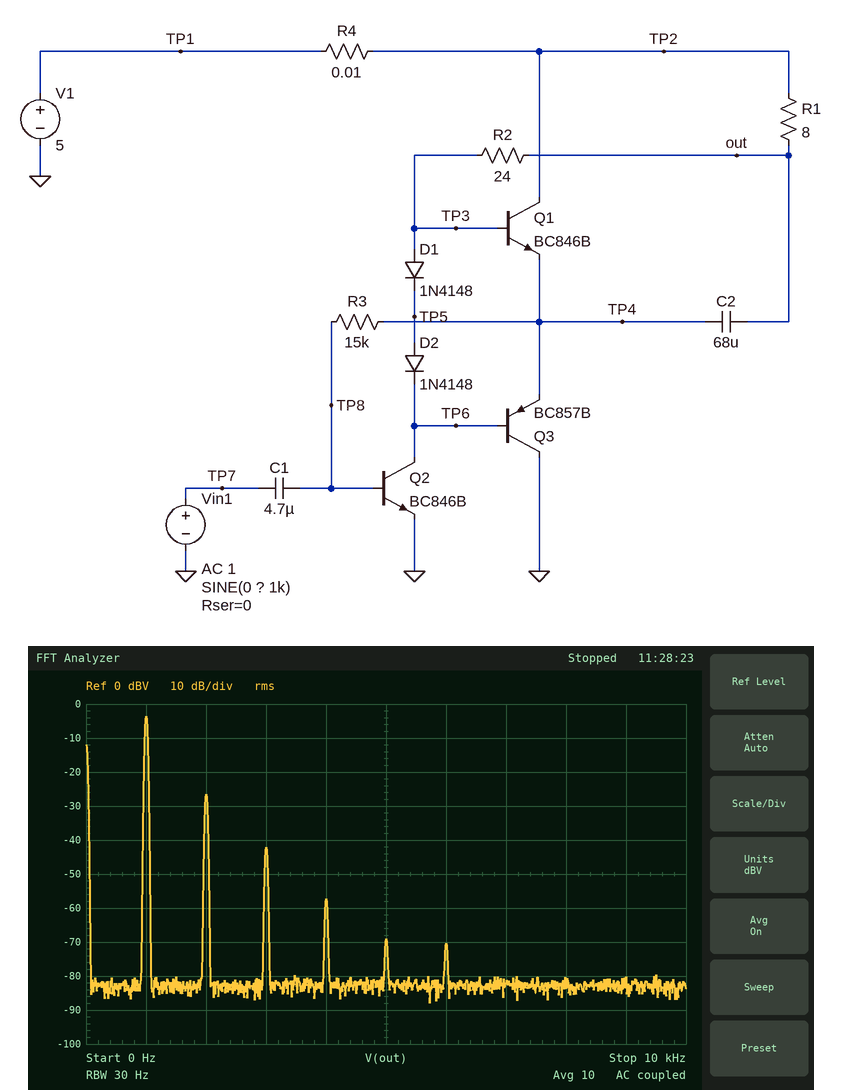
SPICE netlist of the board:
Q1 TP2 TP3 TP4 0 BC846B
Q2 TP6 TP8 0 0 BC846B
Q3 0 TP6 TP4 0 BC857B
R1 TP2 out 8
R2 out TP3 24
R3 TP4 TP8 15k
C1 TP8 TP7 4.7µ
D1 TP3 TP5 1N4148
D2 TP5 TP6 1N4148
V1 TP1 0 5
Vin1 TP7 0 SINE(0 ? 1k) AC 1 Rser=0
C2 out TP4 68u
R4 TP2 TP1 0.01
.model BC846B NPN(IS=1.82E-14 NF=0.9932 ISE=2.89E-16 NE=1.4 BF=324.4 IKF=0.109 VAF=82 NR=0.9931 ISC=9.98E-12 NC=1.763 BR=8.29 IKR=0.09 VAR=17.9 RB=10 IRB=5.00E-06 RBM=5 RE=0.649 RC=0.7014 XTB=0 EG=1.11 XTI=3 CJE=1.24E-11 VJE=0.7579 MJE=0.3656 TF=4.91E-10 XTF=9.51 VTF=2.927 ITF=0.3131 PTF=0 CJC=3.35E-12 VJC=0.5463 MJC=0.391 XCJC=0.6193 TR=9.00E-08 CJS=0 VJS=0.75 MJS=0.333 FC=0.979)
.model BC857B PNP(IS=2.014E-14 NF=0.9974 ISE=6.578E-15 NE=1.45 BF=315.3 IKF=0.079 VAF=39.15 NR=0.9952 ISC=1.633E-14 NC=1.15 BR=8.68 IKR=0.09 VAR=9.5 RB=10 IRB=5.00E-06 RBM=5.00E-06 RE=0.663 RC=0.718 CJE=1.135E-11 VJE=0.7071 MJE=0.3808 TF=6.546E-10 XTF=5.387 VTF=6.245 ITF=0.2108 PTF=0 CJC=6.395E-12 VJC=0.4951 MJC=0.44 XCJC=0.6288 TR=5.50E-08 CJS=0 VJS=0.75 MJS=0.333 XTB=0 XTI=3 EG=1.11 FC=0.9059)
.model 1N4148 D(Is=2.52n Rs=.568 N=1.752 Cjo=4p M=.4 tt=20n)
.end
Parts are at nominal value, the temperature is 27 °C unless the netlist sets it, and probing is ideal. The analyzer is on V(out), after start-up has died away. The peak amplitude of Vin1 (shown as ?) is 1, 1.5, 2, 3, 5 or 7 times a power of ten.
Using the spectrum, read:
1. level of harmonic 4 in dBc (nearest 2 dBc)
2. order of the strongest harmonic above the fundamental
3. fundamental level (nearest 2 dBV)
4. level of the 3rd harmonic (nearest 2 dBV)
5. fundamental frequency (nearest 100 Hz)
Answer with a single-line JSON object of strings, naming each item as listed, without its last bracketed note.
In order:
{"level of harmonic 4 in dBc": "-54 dBc", "order of the strongest harmonic above the fundamental": "2", "fundamental level": "-4 dBV", "level of the 3rd harmonic": "-42 dBV", "fundamental frequency": "1.0 kHz"}
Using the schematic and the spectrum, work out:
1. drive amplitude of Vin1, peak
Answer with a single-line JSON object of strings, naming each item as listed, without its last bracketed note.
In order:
{"drive amplitude of Vin1, peak": "20 mV"}
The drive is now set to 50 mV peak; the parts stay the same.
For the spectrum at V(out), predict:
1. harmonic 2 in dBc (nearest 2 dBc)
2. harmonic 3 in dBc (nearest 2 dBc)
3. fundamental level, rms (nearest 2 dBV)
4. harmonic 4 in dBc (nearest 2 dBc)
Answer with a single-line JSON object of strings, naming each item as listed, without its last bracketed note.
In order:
{"harmonic 2 in dBc": "-14 dBc", "harmonic 3 in dBc": "-24 dBc", "fundamental level, rms": "2 dBV", "harmonic 4 in dBc": "-28 dBc"}
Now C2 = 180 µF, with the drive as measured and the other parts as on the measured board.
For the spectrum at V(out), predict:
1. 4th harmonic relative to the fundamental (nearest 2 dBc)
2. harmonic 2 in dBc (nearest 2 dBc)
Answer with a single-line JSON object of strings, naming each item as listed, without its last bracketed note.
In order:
{"4th harmonic relative to the fundamental": "-42 dBc", "harmonic 2 in dBc": "-24 dBc"}
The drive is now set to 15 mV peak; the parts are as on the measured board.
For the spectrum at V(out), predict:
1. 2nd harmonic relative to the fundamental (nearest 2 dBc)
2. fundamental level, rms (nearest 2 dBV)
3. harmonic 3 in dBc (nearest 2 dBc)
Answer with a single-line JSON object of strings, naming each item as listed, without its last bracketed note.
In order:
{"2nd harmonic relative to the fundamental": "-26 dBc", "fundamental level, rms": "-6 dBV", "harmonic 3 in dBc": "-42 dBc"}
